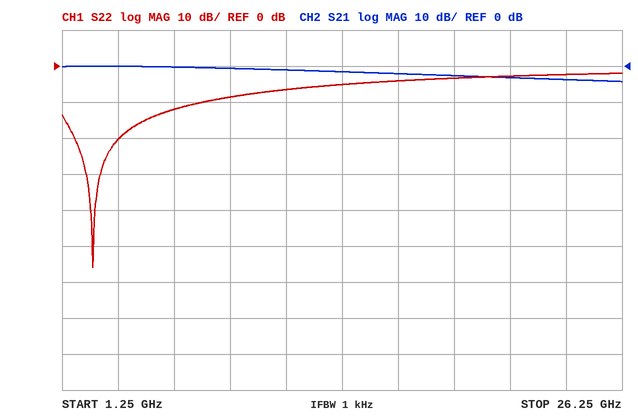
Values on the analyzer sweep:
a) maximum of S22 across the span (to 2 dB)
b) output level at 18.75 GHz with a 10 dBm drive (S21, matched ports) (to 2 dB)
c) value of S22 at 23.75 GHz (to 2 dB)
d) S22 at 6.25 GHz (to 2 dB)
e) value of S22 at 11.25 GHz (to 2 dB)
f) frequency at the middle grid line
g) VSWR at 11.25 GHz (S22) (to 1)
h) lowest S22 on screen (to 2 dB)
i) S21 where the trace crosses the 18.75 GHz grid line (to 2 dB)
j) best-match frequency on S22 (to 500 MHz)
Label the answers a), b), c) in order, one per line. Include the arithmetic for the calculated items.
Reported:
a) -2 dB
b) 10 dBm + (-2 dB) = 8 dBm
c) -2 dB
d) -12 dB
e) -6 dB
f) 13.75 GHz
g) |Γ| = 10^(-6/20) = 0.5012; VSWR = (1 + 0.5012)/(1 − 0.5012) ≈ 3
h) -56 dB
i) -2 dB
j) 2.5 GHz
